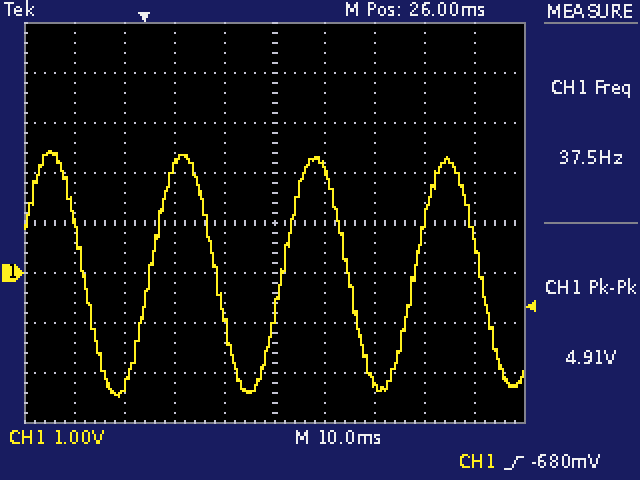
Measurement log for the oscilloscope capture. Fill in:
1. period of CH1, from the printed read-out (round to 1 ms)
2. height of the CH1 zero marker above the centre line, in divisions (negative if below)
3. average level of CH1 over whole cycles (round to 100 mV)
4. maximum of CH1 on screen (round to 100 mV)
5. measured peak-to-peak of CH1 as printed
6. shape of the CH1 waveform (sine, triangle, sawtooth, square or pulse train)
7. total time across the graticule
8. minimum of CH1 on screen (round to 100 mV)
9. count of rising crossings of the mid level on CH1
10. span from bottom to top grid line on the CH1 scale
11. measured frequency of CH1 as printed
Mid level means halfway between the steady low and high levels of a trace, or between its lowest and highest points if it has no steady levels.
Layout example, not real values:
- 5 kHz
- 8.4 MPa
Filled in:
- 27 ms
- -1.0 div
- 0.0 V
- 2.4 V
- 4.91 V
- sine
- 100 ms
- -2.5 V
- 3
- 8 V
- 37.5 Hz
